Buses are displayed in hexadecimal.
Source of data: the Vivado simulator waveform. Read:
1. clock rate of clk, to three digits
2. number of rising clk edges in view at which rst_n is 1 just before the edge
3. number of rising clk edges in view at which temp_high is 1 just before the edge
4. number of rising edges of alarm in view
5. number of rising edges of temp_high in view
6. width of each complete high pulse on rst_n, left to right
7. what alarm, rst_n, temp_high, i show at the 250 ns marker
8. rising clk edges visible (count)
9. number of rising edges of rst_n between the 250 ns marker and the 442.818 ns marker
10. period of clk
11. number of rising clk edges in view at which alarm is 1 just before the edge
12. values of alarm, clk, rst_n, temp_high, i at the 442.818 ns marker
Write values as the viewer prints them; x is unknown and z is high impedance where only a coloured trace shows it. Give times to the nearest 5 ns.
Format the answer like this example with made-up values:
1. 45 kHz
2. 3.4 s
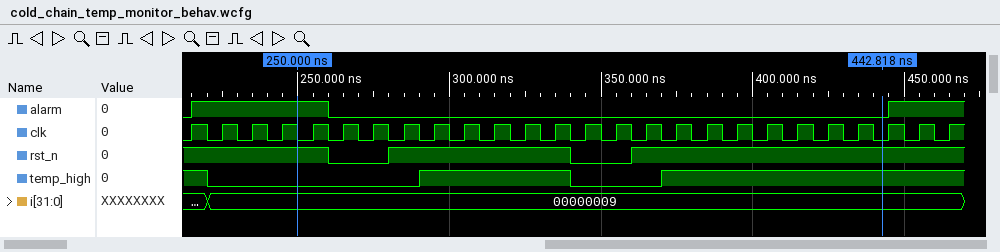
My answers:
1. 100 MHz
2. 22
3. 16
4. 2
5. 2
6. 60 ns
7. alarm=1, rst_n=1, temp_high=0, i=00000009
8. 26
9. 2
10. 10 ns
11. 6
12. alarm=0, clk=0, rst_n=1, temp_high=1, i=00000009
